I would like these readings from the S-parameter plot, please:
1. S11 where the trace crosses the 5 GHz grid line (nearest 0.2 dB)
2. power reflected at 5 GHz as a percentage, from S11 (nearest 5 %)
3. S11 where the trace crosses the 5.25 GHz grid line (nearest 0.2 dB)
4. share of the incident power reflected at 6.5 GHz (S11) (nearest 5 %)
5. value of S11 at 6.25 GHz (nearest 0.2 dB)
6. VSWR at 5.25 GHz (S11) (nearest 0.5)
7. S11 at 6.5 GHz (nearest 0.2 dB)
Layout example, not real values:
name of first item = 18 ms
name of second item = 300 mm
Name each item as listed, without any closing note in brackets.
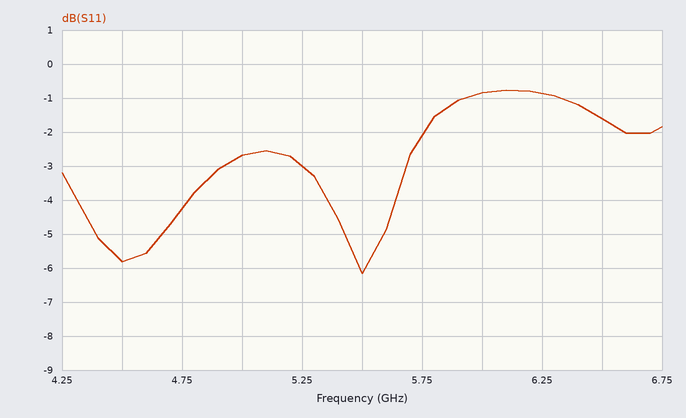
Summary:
S11 where the trace crosses the 5 GHz grid line = -2.6 dB
power reflected at 5 GHz as a percentage, from S11 = 55 %
S11 where the trace crosses the 5.25 GHz grid line = -3.0 dB
share of the incident power reflected at 6.5 GHz (S11) = 70 %
value of S11 at 6.25 GHz = -0.8 dB
VSWR at 5.25 GHz (S11) = 6.0
S11 at 6.5 GHz = -1.6 dB
